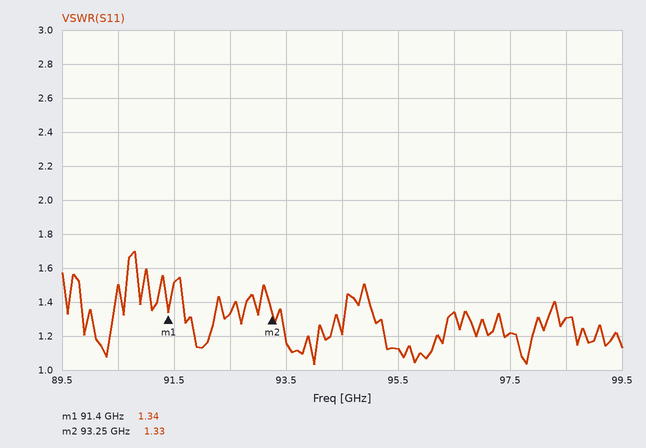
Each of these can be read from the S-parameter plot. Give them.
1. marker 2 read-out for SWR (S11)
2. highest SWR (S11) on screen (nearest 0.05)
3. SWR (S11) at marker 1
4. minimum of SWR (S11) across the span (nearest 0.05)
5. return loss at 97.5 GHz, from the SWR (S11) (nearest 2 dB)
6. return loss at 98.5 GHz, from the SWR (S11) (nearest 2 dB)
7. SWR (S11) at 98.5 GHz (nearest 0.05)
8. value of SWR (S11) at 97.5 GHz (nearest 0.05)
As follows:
1.33
1.70
1.34
1.05
20 dB
18 dB
1.30
1.20
